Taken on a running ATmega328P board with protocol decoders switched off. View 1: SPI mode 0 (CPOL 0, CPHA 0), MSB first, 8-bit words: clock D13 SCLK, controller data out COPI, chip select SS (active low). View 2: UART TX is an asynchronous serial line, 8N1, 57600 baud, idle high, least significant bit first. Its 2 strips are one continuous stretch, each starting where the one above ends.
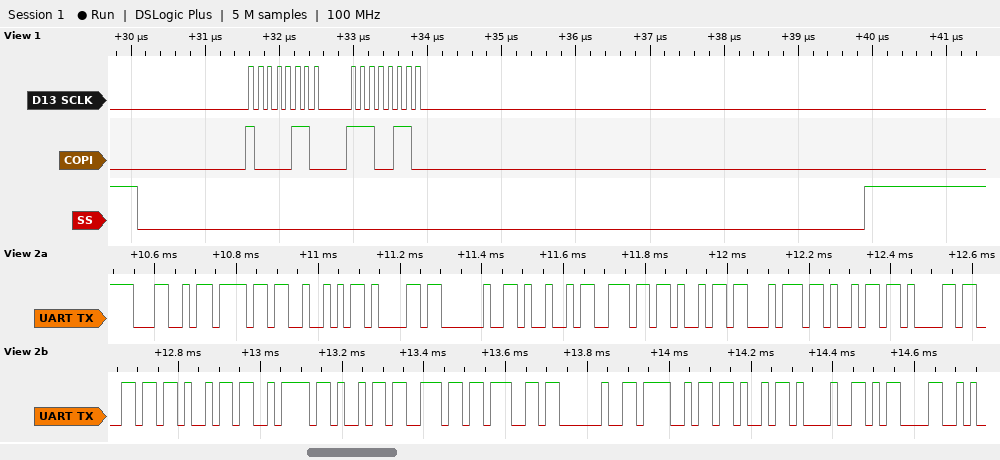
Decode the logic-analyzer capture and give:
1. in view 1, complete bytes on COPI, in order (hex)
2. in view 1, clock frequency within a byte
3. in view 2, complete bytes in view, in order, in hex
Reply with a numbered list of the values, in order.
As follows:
1. 86 E6
2. 8 MHz
3. 4C 6F 52 61 20 49 6E 69 74 69 61 6C 69 7A 69 6E 67 20 4F 4B 21 0D
